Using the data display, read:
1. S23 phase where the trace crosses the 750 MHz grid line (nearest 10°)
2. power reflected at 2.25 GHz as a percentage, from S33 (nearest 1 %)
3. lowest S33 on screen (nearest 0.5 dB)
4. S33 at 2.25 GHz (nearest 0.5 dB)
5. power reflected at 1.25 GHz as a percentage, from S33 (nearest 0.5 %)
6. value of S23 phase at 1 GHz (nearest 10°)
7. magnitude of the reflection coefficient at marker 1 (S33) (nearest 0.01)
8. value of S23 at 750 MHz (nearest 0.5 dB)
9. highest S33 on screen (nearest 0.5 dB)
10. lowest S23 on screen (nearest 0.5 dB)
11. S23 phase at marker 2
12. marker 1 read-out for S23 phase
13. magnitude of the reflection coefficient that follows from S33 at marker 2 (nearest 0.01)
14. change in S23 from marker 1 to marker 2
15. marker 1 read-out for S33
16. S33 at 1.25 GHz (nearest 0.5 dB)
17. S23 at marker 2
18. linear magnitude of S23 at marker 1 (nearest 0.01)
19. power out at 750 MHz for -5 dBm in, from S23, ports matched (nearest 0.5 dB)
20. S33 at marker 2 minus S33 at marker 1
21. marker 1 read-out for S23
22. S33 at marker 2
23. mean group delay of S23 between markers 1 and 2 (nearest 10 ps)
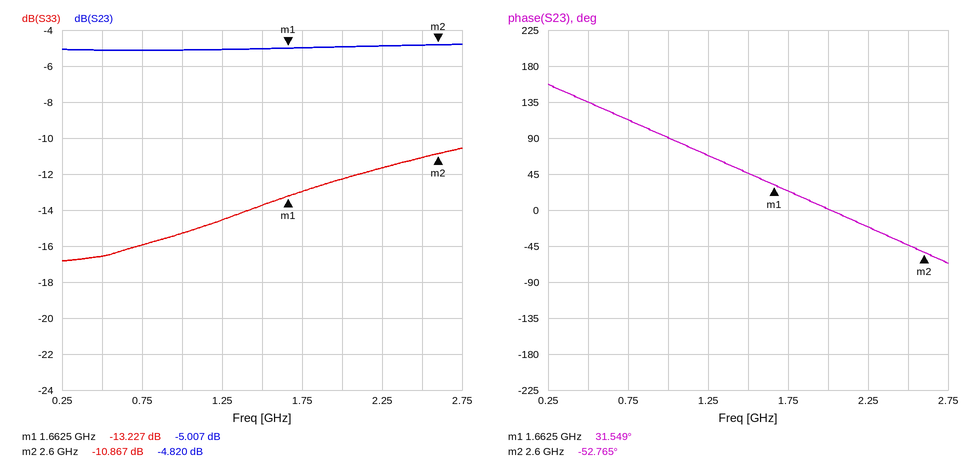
110°
7 %
-17.0 dB
-11.5 dB
3.5 %
90°
0.22
-5.0 dB
-10.5 dB
-5.0 dB
-52.765°
31.549°
0.29
0.187 dB
-13.227 dB
-14.5 dB
-4.820 dB
0.56
-10.0 dBm
2.360 dB
-5.007 dB
-10.867 dB
250 ps
